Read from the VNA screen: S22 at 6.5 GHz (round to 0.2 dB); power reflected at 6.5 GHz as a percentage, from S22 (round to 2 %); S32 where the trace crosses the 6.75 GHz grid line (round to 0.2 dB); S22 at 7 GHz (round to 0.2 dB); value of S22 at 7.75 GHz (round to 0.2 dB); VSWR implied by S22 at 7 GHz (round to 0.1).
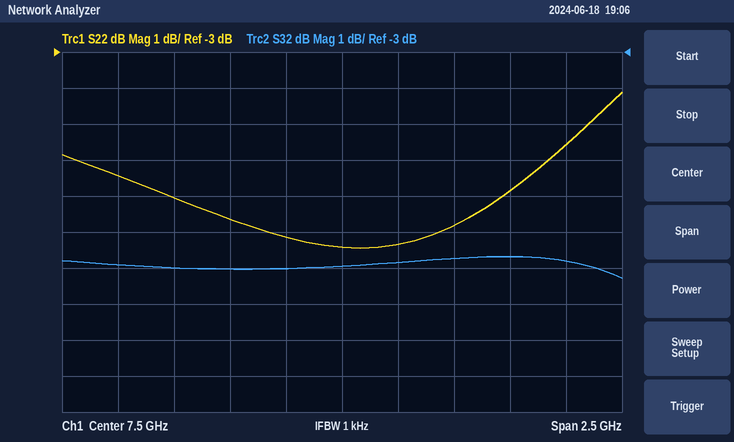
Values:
-6.4 dB
22 %
-9.0 dB
-7.6 dB
-8.4 dB
2.4
